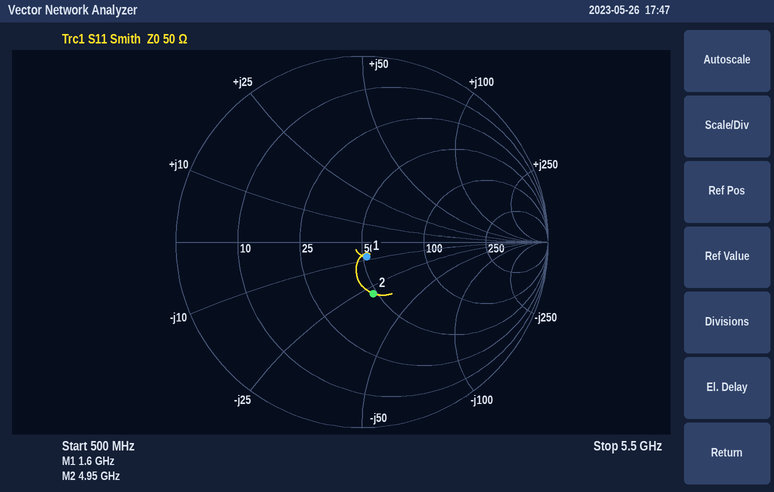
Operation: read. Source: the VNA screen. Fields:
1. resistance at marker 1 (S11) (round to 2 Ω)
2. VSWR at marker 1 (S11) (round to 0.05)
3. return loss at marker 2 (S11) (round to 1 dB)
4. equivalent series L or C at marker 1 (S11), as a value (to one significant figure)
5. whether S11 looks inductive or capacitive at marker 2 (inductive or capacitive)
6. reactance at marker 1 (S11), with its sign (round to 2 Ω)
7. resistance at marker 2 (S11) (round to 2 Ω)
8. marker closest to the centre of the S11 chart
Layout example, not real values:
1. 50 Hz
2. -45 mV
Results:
1. 52 Ω
2. 1.20
3. 11 dB
4. 10 pF
5. capacitive
6. -8 Ω
7. 48 Ω
8. marker 1
